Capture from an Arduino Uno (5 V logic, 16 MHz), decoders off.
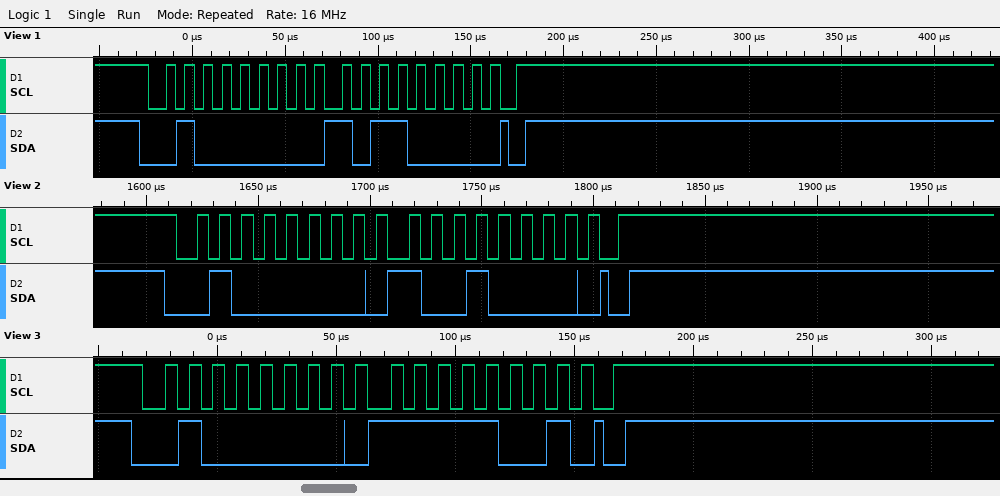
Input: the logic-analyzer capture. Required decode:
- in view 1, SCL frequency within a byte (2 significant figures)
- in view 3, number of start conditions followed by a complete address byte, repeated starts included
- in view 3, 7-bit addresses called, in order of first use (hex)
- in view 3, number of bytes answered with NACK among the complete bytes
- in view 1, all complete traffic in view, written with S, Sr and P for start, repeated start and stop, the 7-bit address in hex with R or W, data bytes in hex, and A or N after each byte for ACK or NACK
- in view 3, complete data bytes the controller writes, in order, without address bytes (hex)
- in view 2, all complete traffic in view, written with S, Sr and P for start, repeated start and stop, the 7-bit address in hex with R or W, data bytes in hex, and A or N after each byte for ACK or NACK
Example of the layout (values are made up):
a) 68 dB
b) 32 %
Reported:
a) 100 kHz
b) 1
c) 0x20
d) 0
e) S 20W A B0 A P
f) F9
g) S 20W A 90 A P
